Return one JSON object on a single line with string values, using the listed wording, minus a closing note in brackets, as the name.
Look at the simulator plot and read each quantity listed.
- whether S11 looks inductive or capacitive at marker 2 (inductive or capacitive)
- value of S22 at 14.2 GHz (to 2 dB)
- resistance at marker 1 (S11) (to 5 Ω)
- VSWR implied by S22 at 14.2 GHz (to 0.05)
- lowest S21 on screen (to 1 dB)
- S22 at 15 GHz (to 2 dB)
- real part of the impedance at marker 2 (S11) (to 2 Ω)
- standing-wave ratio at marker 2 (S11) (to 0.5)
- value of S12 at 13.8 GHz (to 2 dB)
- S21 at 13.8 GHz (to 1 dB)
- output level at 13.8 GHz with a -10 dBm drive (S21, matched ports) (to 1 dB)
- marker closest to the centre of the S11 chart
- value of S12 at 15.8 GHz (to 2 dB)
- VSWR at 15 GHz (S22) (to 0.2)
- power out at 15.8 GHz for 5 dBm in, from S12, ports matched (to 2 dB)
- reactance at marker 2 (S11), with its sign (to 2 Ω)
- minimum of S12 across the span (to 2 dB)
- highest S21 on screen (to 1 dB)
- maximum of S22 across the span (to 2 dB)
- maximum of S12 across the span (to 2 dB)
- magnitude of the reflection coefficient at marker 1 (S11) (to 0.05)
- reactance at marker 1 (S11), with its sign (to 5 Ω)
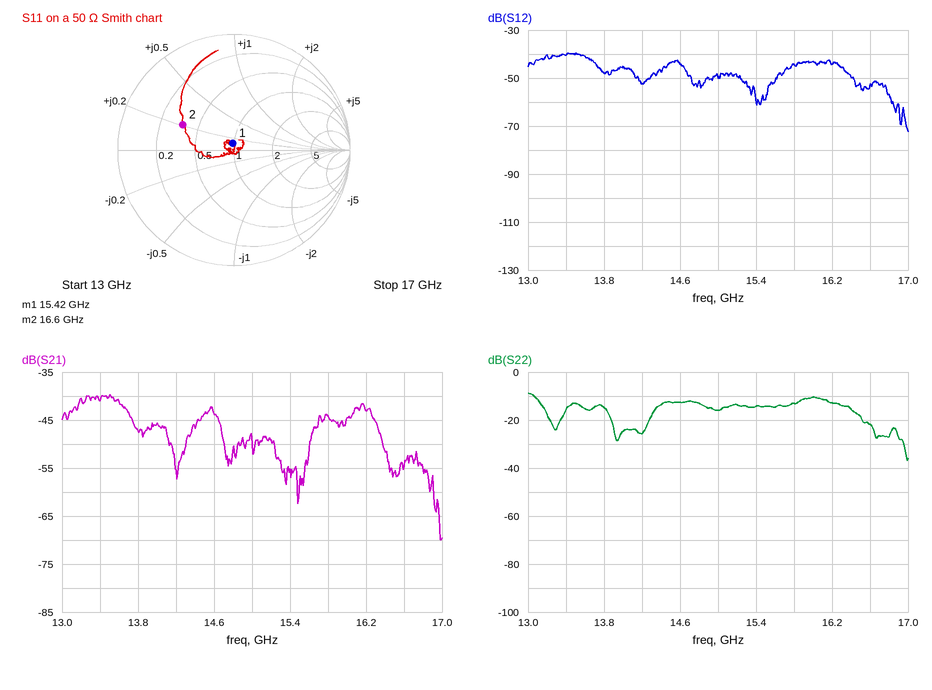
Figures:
{"whether S11 looks inductive or capacitive at marker 2": "inductive", "value of S22 at 14.2 GHz": "-26 dB", "resistance at marker 1 (S11)": "50 Ω", "VSWR implied by S22 at 14.2 GHz": "1.10", "lowest S21 on screen": "-70 dB", "S22 at 15 GHz": "-16 dB", "real part of the impedance at marker 2 (S11)": "18 Ω", "standing-wave ratio at marker 2 (S11)": "3.0", "value of S12 at 13.8 GHz": "-48 dB", "S21 at 13.8 GHz": "-47 dB", "output level at 13.8 GHz with a -10 dBm drive (S21, matched ports)": "-57 dBm", "marker closest to the centre of the S11 chart": "marker 1", "value of S12 at 15.8 GHz": "-44 dB", "VSWR at 15 GHz (S22)": "1.4", "power out at 15.8 GHz for 5 dBm in, from S12, ports matched": "-40 dBm", "reactance at marker 2 (S11), with its sign": "+10 Ω", "minimum of S12 across the span": "-72 dB", "highest S21 on screen": "-40 dB", "maximum of S22 across the span": "-8 dB", "maximum of S12 across the span": "-40 dB", "magnitude of the reflection coefficient at marker 1 (S11)": "0.05", "reactance at marker 1 (S11), with its sign": "+5 Ω"}
